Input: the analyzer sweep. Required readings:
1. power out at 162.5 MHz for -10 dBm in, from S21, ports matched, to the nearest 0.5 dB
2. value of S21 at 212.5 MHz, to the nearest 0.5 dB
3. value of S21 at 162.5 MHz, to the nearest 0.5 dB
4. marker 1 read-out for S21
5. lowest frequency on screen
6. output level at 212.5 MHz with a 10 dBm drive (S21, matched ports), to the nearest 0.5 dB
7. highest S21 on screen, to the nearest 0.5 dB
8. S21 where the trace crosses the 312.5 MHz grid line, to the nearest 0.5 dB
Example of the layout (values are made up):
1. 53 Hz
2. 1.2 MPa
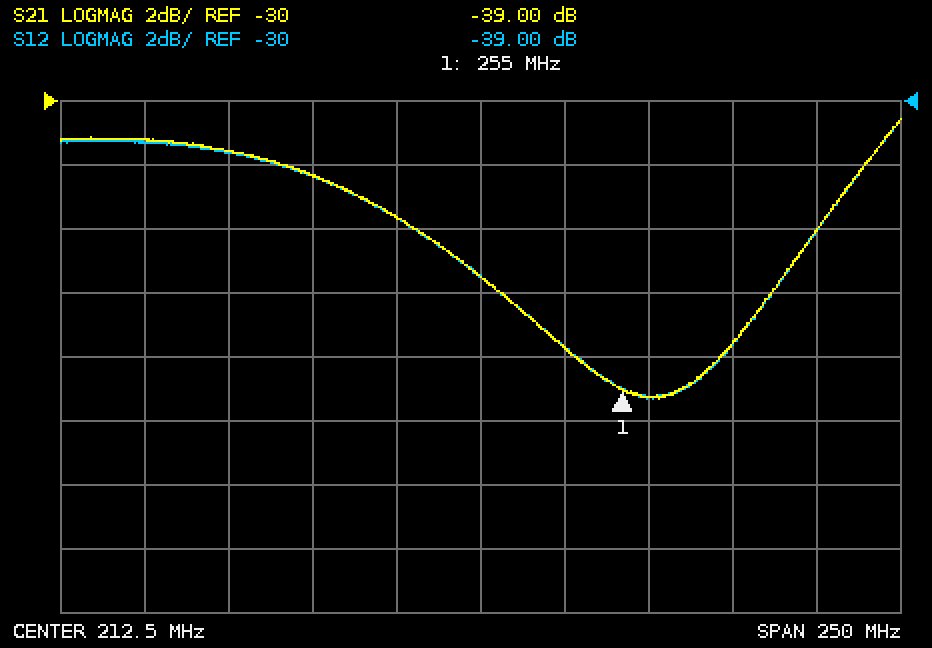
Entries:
1. -42.5 dBm
2. -35.5 dB
3. -32.5 dB
4. -39.00 dB
5. 87.5 MHz
6. -25.5 dBm
7. -30.5 dB
8. -34.0 dB
